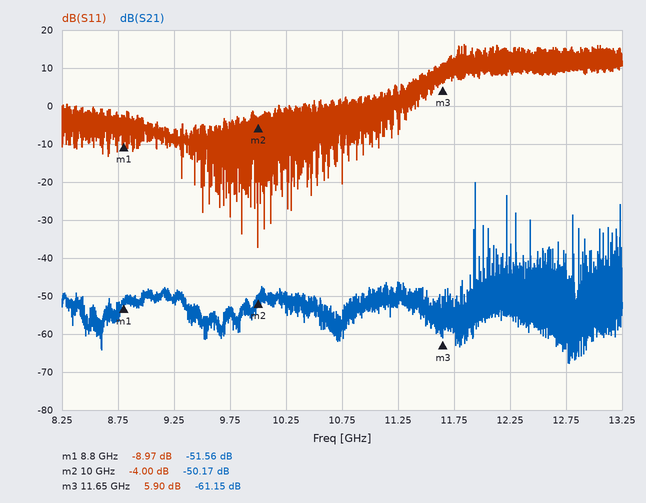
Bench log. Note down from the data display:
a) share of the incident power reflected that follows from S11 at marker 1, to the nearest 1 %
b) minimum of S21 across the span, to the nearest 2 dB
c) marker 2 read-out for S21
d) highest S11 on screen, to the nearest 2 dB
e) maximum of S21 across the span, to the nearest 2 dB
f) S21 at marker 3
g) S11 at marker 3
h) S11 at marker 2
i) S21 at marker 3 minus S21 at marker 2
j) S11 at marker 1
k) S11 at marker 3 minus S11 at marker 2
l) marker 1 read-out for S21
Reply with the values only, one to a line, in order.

13 %
-68 dB
-50.17 dB
16 dB
-20 dB
-61.15 dB
5.90 dB
-4.00 dB
-10.98 dB
-8.97 dB
9.90 dB
-51.56 dB
